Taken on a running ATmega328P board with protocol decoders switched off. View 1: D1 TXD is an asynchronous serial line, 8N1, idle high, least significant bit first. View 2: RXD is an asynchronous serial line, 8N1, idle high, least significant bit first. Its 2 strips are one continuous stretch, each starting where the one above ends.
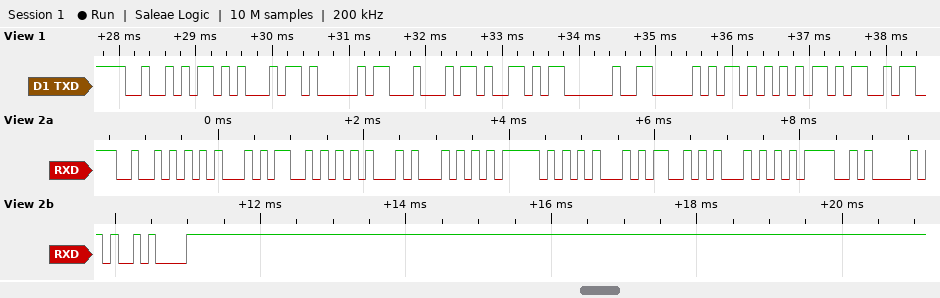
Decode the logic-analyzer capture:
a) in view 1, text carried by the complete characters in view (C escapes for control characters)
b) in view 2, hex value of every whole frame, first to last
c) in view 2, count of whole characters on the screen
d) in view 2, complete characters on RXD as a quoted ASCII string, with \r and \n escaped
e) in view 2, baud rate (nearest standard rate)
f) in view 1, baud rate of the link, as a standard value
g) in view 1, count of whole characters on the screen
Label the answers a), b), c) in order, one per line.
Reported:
a) "READY PUM"
b) 52 45 53 45 54 5F 45 53 54 4F 50 0A
c) 12
d) "RESET_ESTOP\n"
e) 9600 baud
f) 9600 baud
g) 9
